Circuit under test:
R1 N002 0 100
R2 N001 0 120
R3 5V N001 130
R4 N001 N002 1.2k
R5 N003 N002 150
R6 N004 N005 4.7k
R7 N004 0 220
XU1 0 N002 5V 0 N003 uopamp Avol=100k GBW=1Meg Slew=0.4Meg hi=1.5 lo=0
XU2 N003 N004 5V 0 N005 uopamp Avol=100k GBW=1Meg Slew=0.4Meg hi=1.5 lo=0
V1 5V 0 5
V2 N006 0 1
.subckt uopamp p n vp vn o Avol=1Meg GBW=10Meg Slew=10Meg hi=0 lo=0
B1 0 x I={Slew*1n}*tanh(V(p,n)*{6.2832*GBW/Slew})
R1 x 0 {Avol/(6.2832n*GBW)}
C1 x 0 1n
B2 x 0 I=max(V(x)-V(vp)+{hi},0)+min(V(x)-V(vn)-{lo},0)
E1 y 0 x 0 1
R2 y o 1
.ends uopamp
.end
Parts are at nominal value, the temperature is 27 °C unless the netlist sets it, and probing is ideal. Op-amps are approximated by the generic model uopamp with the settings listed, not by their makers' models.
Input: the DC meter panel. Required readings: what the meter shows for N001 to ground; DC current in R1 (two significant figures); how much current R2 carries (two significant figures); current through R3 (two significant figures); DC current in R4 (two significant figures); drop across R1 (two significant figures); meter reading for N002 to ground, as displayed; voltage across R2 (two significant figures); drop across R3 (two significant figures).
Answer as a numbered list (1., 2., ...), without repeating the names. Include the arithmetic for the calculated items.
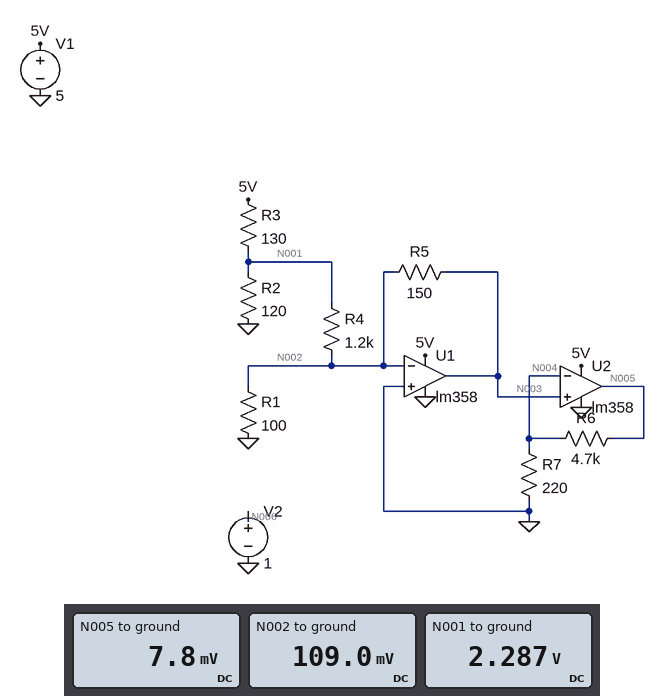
1. 2.287 V
2. (109 mV) / 100 Ω = 1.1 mA
3. (2.287 V) / 120 Ω = 19 mA
4. (5 V - 2.287 V) / 130 Ω = 21 mA
5. (2.287 V - 109 mV) / 1.2 kΩ = 1.8 mA
6. 109 mV = 110 mV
7. 109.0 mV
8. 2.287 V = 2.3 V
9. 5 V - 2.287 V = 2.7 V
